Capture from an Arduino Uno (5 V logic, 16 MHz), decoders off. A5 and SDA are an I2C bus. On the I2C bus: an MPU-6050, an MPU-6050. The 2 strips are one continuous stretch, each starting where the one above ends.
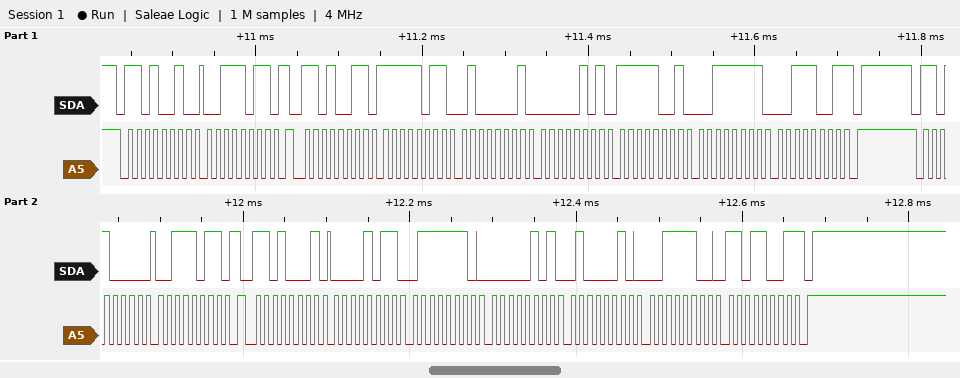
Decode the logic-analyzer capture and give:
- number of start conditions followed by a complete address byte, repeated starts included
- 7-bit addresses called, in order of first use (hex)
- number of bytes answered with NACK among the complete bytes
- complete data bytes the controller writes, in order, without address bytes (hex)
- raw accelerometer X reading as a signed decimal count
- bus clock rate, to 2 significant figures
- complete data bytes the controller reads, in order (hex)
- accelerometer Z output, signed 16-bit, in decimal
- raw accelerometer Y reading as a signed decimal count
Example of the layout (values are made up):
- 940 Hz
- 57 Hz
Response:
- 4
- 0x69 0x68
- 2
- 3B 3B
- -1215
- 100 kHz
- FB 41 05 F9 3F 39 0B 7E 05 42 3C D9
- 16185
- 1529
